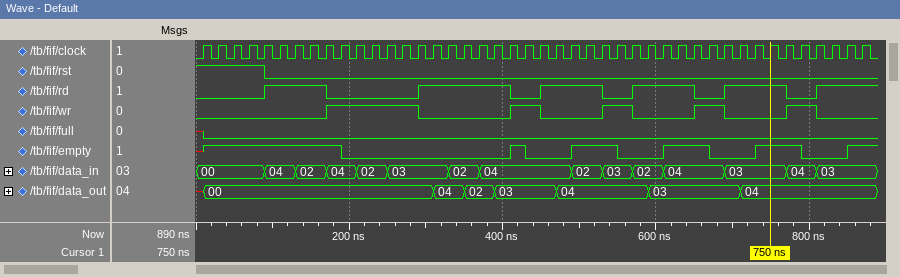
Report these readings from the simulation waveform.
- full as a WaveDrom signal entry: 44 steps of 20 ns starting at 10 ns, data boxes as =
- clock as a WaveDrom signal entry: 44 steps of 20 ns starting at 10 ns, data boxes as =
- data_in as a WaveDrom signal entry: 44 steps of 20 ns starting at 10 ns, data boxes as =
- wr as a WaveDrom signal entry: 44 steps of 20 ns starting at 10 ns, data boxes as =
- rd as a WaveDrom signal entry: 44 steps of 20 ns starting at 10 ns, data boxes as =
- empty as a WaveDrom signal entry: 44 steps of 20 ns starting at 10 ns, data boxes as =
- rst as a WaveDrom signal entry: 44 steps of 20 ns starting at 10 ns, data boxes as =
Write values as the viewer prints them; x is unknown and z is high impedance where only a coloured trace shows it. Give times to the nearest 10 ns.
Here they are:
{name: 'full', wave: '0...........................................'}
{name: 'clock', wave: 'p...........................................'}
{name: 'data_in', wave: '=...=.=.=.=.=...=.=.....=.=.=.=...=...=.=...', data: '00 04 02 04 02 03 02 04 02 03 02 04 03 04 03'}
{name: 'wr', wave: '0.......1.....0.....1.0...1.0...1.0...1.0...'}
{name: 'rd', wave: '0...1...0.....1.....0.1...0.1...0.1...0.1...'}
{name: 'empty', wave: '1........0..........10..1..0..1..0..1..0..1.'}
{name: 'rst', wave: '1...0.......................................'}
